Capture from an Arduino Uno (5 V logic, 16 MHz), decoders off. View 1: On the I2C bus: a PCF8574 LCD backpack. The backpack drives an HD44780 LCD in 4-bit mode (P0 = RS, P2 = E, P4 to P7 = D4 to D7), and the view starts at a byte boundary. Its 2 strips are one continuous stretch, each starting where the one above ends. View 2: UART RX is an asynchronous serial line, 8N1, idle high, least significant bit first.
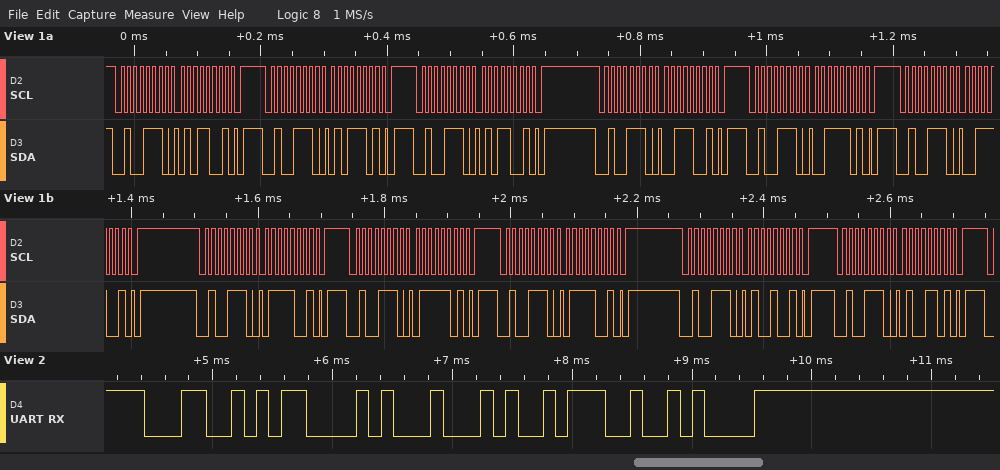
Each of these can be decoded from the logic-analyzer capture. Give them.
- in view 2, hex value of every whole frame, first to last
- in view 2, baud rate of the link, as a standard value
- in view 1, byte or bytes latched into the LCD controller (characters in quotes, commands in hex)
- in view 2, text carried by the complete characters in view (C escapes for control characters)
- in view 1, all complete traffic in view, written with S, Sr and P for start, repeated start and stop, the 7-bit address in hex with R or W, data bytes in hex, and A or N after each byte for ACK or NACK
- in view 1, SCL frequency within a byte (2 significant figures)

4C 43 44 3A 0A
9600 baud
'S'
"LCD:\n"
S 27W A 59 A P S 27W A 5D A P S 27W A 59 A P S 27W A 39 A P S 27W A 3D A P S 27W A 39 A P S 27W A 79 A P S 27W A 7D A P S 27W A 79 A P S 27W A 49 A P S 27W A 4D A P
100 kHz
